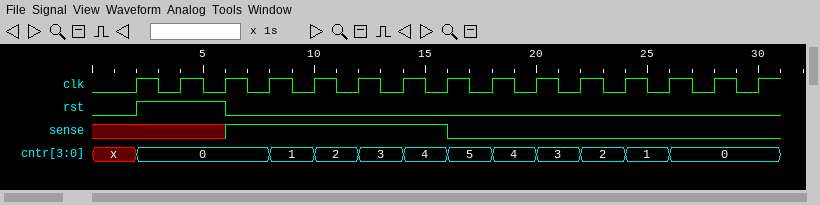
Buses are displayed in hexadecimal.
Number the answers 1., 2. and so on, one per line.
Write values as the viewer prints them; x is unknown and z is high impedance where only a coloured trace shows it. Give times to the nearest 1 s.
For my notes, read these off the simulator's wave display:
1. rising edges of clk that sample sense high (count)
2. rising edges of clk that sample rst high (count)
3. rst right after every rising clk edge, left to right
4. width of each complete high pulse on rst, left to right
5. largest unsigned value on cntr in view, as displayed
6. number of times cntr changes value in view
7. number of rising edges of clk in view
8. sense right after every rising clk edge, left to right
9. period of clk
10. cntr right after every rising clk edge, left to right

1. 5
2. 2
3. 1 1 0 0 0 0 0 0 0 0 0 0 0 0 0
4. 4 s
5. 5
6. 11
7. 15
8. x x 1 1 1 1 1 0 0 0 0 0 0 0 0
9. 2 s
10. 0, 0, 0, 1, 2, 3, 4, 5, 4, 3, 2, 1, 0, 0, 0
